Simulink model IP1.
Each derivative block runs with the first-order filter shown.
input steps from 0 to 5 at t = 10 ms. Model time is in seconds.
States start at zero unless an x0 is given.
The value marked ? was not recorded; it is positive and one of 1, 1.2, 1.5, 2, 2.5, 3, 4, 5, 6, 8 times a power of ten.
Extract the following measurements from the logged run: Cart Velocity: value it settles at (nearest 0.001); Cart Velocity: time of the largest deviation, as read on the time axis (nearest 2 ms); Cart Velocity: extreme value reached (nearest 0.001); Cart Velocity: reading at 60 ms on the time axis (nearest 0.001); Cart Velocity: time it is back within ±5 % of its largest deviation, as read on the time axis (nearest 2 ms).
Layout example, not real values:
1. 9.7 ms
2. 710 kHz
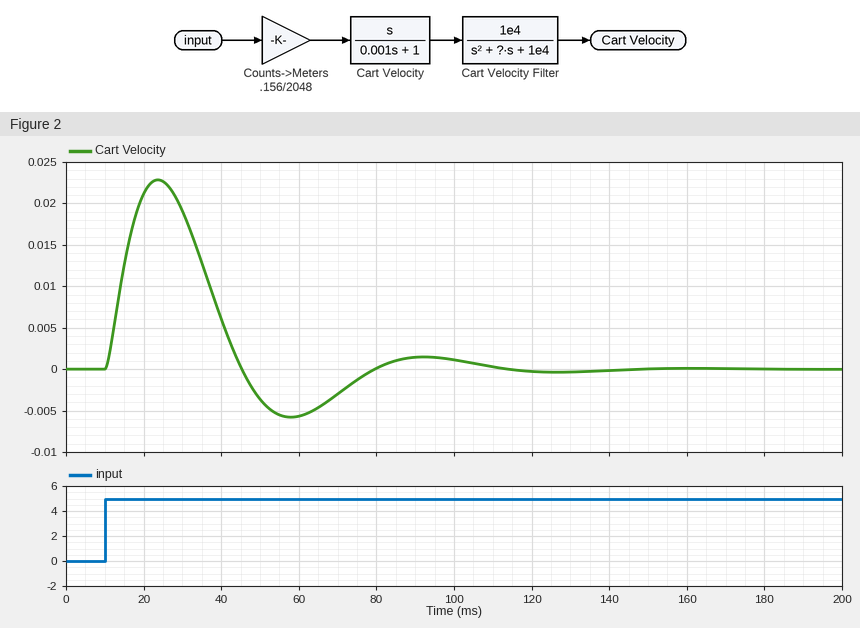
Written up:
1. 0.000
2. 24 ms
3. 0.023
4. -0.006
5. 100 ms
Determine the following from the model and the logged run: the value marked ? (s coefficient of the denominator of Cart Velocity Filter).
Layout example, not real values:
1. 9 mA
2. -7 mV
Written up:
1. 80
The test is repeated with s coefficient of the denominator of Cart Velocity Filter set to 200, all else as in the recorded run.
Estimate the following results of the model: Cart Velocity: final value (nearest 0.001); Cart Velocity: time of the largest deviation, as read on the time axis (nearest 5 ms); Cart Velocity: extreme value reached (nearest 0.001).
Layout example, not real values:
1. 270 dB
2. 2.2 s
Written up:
1. 0.000
2. 20 ms
3. 0.014
